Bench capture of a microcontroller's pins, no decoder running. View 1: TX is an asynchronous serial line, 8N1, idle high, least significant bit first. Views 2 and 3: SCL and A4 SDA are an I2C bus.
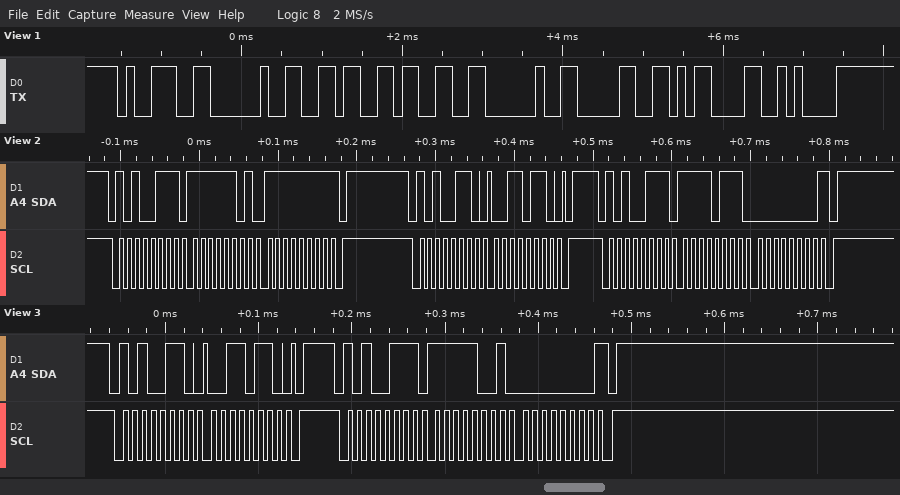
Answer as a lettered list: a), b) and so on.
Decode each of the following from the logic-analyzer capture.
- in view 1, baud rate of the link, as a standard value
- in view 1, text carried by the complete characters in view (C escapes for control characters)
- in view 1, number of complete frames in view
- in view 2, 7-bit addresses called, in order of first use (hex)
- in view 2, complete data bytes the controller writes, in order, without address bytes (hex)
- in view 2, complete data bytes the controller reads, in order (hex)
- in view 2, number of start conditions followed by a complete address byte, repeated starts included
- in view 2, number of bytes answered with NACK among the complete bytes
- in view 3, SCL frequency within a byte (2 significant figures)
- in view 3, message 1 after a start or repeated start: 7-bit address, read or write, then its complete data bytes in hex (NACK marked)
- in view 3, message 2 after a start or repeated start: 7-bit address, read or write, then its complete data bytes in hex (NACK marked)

a) 9600 baud
b) "9 63 0\r\n"
c) 8
d) 0x53
e) 36
f) FD FF F7 00
g) 3
h) 2
i) 100 kHz
j) 0x53 write: 36
k) 0x53 read: F9 00 NACK
